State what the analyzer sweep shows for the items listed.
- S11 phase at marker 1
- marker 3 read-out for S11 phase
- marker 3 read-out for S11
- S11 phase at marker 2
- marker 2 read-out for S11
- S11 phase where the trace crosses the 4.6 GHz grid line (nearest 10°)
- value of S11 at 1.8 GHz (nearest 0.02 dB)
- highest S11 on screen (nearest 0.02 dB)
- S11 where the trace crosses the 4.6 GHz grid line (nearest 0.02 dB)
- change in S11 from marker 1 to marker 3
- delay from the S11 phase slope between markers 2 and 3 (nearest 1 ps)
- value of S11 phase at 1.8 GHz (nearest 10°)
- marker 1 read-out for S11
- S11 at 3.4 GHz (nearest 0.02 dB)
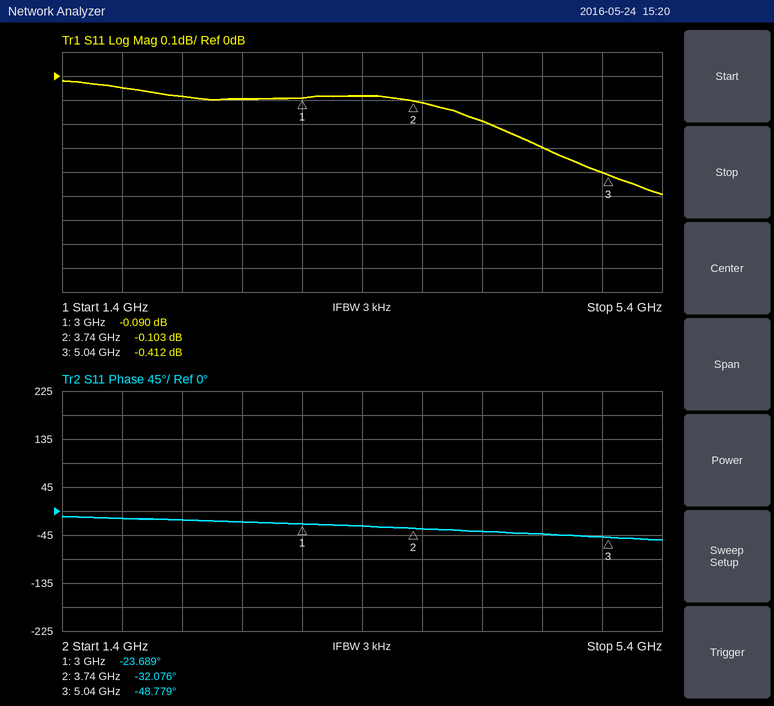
-23.689°
-48.779°
-0.412 dB
-32.076°
-0.103 dB
-40°
-0.04 dB
-0.02 dB
-0.30 dB
-0.322 dB
36 ps
-10°
-0.090 dB
-0.08 dB
